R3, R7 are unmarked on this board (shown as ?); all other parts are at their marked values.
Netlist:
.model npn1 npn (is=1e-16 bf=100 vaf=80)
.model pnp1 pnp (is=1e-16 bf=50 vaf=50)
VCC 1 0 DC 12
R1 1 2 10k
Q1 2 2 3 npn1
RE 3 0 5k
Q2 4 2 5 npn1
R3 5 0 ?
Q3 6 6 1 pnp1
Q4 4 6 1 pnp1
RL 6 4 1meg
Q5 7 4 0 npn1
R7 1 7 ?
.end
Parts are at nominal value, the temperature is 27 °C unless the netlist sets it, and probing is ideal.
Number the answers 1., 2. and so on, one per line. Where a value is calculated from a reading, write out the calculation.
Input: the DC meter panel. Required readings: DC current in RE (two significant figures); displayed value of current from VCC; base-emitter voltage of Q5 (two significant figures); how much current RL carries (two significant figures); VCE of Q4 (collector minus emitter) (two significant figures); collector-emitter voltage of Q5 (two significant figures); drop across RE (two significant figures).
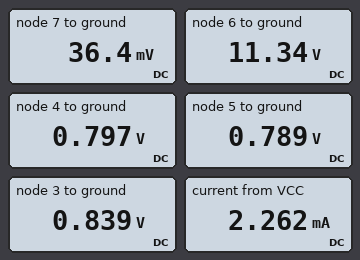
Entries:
1. (839 mV) / 5 kΩ = 170 µA
2. 2.262 mA
3. 797 mV = 800 mV
4. (11.34 V - 797 mV) / 1 MΩ = 11 µA
5. 797 mV - 12 V = -11 V
6. 36.4 mV = 36 mV
7. 839 mV = 840 mV
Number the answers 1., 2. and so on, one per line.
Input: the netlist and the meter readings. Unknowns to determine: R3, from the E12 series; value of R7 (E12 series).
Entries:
1. 2.7 kΩ
2. 10 kΩ
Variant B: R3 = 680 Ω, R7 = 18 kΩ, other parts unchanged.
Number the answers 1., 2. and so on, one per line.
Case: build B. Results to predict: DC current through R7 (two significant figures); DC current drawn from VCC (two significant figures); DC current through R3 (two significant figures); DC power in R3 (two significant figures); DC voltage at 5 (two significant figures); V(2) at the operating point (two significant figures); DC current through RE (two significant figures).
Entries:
1. 12 µA
2. 1.1 mA
3. 940 µA
4. 600 µW
5. 640 mV
6. 1.4 V
7. 140 µA
